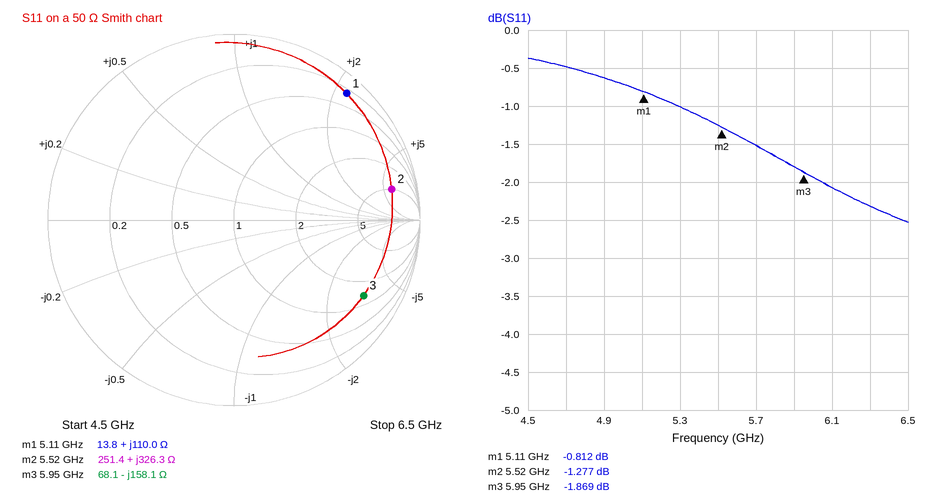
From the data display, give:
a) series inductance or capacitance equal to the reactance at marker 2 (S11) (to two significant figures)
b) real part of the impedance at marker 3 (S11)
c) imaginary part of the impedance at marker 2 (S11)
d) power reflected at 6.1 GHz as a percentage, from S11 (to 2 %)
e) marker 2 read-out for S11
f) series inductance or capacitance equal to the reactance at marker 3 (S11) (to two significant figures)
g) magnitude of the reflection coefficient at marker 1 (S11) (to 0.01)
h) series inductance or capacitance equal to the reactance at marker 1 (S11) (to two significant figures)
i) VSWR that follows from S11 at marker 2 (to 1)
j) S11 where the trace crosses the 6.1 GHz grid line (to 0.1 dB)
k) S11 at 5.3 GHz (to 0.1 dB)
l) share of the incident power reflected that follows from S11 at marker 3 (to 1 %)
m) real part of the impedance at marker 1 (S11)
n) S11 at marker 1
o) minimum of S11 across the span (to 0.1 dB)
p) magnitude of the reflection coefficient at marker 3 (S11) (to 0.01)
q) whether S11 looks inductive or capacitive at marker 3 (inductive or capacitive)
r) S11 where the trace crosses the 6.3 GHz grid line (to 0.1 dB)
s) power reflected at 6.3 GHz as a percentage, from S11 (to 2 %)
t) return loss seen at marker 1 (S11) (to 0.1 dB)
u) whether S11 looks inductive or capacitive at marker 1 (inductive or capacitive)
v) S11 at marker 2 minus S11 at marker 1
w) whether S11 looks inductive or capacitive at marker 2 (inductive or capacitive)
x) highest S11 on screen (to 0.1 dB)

9.4 nH
68.1 Ω
+326.3 Ω
62 %
-1.277 dB
170 fF
0.91
3.4 nH
14
-2.1 dB
-1.0 dB
65 %
13.8 Ω
-0.812 dB
-2.5 dB
0.81
capacitive
-2.3 dB
58 %
0.8 dB
inductive
-0.465 dB
inductive
-0.4 dB
